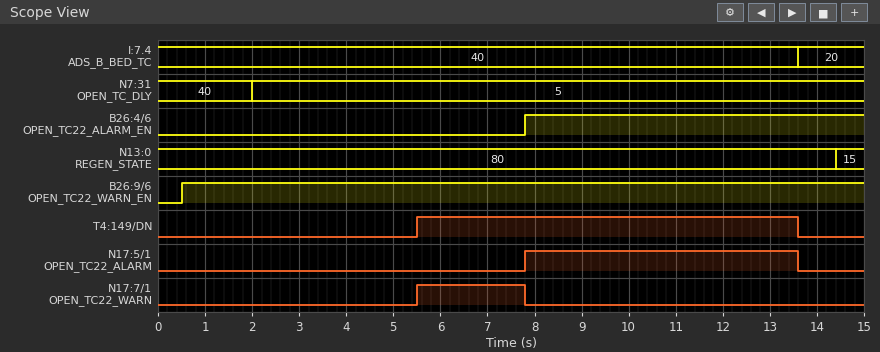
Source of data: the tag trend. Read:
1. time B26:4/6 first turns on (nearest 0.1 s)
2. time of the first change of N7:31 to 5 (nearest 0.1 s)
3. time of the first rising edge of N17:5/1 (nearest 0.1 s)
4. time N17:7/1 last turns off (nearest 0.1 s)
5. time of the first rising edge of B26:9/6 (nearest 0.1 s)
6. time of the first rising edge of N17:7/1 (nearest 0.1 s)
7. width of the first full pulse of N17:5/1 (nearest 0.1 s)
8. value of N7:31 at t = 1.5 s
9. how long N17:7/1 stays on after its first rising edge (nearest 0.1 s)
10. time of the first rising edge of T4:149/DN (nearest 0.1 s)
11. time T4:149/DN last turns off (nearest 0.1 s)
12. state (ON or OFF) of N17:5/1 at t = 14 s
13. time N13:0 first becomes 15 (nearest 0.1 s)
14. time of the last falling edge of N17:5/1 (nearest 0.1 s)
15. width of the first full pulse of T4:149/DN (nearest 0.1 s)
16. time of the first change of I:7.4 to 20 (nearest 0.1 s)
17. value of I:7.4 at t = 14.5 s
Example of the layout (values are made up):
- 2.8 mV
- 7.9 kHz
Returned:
- 7.8 s
- 2.0 s
- 7.8 s
- 7.8 s
- 0.5 s
- 5.5 s
- 5.8 s
- 40
- 2.3 s
- 5.5 s
- 13.6 s
- OFF
- 14.4 s
- 13.6 s
- 8.1 s
- 13.6 s
- 20
